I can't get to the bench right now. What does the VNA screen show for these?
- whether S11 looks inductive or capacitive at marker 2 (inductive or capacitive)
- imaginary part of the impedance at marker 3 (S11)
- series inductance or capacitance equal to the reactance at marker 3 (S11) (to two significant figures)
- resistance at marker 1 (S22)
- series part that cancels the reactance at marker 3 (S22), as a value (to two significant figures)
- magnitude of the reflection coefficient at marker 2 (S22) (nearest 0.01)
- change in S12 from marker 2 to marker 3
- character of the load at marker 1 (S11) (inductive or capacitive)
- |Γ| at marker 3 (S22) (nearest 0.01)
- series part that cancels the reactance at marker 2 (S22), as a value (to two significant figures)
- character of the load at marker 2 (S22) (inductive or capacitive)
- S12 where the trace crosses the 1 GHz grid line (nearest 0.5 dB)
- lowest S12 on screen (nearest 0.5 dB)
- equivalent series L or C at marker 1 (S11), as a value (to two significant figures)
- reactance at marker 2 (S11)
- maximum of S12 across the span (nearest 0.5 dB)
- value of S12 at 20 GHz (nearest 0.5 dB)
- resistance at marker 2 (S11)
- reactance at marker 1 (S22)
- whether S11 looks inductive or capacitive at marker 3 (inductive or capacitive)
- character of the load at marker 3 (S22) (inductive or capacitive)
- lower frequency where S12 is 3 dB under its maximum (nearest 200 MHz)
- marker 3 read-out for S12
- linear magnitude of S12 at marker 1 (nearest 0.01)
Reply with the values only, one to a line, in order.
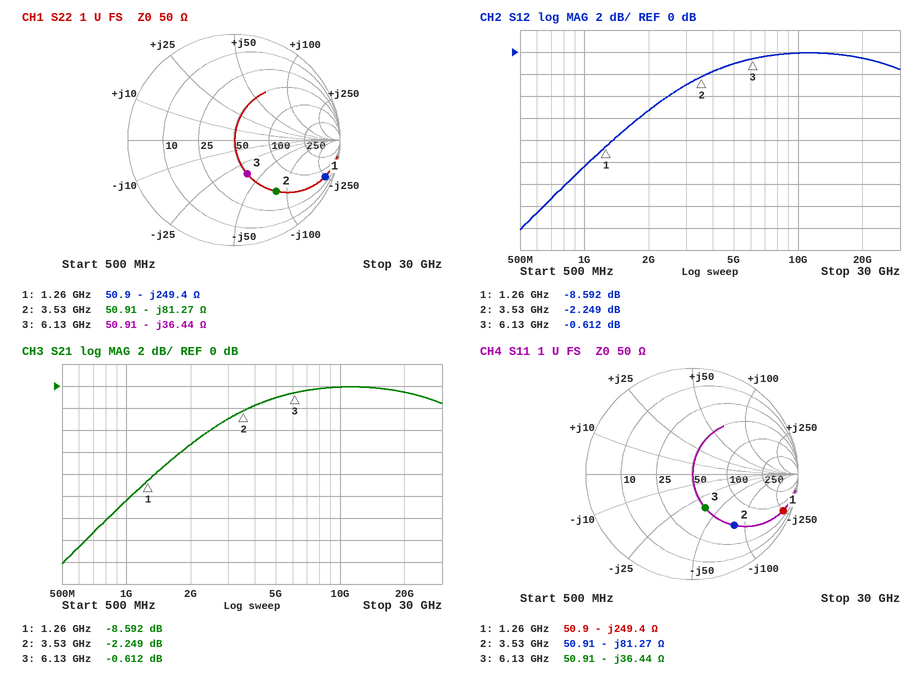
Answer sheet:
capacitive
-36.44 Ω
710 fF
50.9 Ω
950 pH
0.63
1.637 dB
capacitive
0.34
3.7 nH
capacitive
-10.5 dB
-16.0 dB
510 fF
-81.27 Ω
0.0 dB
-0.5 dB
50.91 Ω
-249.4 Ω
capacitive
capacitive
3.0 GHz
-0.612 dB
0.37
